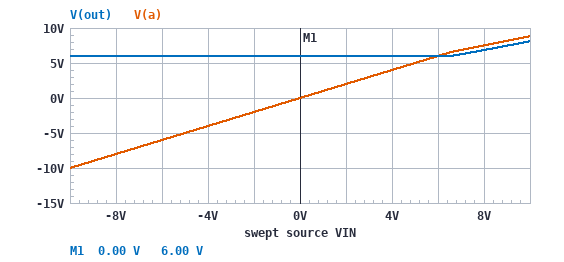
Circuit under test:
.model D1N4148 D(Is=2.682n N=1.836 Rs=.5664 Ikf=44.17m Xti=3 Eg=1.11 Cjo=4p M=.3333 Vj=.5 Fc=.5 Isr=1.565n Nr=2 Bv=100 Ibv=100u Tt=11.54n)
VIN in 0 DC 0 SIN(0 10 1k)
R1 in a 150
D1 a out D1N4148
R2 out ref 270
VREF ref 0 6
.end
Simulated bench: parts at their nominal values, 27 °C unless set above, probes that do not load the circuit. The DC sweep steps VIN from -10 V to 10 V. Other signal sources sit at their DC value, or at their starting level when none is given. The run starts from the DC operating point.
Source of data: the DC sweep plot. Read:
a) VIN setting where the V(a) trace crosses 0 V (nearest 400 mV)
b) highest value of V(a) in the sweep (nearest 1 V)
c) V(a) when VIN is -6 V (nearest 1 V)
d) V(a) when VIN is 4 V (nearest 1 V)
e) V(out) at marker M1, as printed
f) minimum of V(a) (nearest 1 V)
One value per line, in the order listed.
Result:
0 V
9 V
-6 V
4 V
6.00 V
-10 V
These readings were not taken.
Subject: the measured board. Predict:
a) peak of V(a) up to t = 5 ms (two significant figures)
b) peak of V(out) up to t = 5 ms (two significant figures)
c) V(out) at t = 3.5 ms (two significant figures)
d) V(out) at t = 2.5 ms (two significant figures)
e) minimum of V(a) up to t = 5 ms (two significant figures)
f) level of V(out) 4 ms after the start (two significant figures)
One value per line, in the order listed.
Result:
8.8 V
8.1 V
6.0 V
6.0 V
-10 V
6.0 V
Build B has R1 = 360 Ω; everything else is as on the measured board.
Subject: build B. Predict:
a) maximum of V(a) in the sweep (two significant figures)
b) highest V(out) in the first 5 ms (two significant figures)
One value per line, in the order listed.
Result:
8.1 V
7.4 V
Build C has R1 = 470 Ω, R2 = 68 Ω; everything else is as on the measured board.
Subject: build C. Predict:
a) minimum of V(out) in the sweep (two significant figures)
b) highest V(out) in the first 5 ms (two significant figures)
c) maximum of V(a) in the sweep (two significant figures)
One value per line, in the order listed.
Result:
6.0 V
6.4 V
7.1 V
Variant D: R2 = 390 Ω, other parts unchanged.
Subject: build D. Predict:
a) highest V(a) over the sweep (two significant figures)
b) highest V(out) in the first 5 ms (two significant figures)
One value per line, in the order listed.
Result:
9.1 V
8.4 V
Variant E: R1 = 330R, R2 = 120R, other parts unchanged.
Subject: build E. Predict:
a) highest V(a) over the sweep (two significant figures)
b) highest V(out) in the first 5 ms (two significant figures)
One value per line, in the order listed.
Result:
7.6 V
6.9 V
